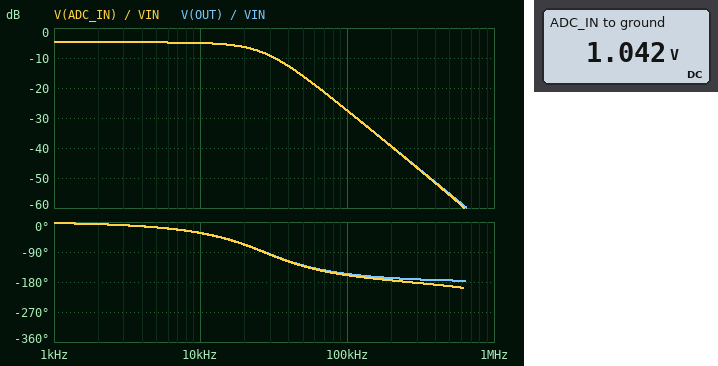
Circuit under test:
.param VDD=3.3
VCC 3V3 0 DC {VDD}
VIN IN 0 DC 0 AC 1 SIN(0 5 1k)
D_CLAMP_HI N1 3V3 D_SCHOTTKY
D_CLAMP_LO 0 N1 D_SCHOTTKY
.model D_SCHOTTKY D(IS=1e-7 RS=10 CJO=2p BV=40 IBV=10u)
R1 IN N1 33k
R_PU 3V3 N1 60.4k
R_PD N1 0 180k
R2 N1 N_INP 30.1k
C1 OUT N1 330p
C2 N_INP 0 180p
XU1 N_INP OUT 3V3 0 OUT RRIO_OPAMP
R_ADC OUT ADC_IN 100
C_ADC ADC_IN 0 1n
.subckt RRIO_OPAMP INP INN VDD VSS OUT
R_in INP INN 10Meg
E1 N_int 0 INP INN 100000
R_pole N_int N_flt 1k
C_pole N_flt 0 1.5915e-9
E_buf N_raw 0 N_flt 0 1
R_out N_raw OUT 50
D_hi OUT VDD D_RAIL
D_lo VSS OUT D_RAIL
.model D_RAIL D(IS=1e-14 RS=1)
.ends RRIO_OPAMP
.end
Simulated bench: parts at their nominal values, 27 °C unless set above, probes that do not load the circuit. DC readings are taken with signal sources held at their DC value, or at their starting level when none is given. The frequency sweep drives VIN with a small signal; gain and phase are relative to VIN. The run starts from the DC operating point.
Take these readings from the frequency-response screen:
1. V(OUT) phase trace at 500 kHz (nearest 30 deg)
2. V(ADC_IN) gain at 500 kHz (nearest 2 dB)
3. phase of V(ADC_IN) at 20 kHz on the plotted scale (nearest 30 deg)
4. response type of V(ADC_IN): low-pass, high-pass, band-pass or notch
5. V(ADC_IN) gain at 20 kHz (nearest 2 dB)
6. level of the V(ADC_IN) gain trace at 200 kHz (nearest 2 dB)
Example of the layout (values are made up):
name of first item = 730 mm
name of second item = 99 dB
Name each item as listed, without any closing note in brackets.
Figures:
V(OUT) phase trace at 500 kHz = -180 deg
V(ADC_IN) gain at 500 kHz = -56 dB
phase of V(ADC_IN) at 20 kHz on the plotted scale = -60 deg
response type of V(ADC_IN): low-pass, high-pass, band-pass or notch = low-pass
V(ADC_IN) gain at 20 kHz = -6 dB
level of the V(ADC_IN) gain trace at 200 kHz = -40 dB
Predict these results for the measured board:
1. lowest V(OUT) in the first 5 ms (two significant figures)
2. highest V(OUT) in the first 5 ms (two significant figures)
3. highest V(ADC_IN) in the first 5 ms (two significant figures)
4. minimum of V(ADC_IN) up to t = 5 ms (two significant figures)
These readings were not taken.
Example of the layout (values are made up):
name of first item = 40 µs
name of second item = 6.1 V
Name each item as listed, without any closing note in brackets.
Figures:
lowest V(OUT) in the first 5 ms = -180 mV
highest V(OUT) in the first 5 ms = 3.4 V
highest V(ADC_IN) in the first 5 ms = 3.4 V
minimum of V(ADC_IN) up to t = 5 ms = -180 mV
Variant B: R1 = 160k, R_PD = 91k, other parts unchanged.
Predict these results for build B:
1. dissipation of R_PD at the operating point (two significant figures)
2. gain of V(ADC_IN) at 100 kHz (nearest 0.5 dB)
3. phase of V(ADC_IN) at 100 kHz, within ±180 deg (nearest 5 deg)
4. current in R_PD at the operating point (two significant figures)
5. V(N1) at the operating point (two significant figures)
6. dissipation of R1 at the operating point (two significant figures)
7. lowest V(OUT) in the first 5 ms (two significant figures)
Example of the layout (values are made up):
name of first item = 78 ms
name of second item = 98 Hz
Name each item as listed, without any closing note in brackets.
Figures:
dissipation of R_PD at the operating point = 29 µW
gain of V(ADC_IN) at 100 kHz = -41.0 dB
phase of V(ADC_IN) at 100 kHz, within ±180 deg = -165 deg
current in R_PD at the operating point = 18 µA
V(N1) at the operating point = 1.6 V
dissipation of R1 at the operating point = 16 µW
lowest V(OUT) in the first 5 ms = 690 mV
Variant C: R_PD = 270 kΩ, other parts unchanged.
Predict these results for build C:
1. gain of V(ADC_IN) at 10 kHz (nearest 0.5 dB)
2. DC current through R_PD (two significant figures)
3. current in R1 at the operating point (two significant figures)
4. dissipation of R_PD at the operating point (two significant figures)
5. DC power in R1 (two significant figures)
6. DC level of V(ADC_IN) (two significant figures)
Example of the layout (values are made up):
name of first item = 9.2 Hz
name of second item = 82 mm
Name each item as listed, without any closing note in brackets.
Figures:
gain of V(ADC_IN) at 10 kHz = -4.5 dB
DC current through R_PD = 4.0 µA
current in R1 at the operating point = 33 µA
dissipation of R_PD at the operating point = 4.3 µW
DC power in R1 = 35 µW
DC level of V(ADC_IN) = 1.1 V
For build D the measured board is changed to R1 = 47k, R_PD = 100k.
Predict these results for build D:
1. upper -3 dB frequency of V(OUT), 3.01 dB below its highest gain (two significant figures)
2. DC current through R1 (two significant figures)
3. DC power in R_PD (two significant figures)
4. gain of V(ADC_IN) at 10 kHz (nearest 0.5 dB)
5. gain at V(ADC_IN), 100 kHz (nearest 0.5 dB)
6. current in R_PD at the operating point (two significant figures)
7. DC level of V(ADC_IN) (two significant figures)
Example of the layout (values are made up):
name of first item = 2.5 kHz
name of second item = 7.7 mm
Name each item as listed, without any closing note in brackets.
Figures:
upper -3 dB frequency of V(OUT), 3.01 dB below its highest gain = 24 kHz
DC current through R1 = 24 µA
DC power in R_PD = 13 µW
gain of V(ADC_IN) at 10 kHz = -7.5 dB
gain at V(ADC_IN), 100 kHz = -30.5 dB
current in R_PD at the operating point = 11 µA
DC level of V(ADC_IN) = 1.1 V
